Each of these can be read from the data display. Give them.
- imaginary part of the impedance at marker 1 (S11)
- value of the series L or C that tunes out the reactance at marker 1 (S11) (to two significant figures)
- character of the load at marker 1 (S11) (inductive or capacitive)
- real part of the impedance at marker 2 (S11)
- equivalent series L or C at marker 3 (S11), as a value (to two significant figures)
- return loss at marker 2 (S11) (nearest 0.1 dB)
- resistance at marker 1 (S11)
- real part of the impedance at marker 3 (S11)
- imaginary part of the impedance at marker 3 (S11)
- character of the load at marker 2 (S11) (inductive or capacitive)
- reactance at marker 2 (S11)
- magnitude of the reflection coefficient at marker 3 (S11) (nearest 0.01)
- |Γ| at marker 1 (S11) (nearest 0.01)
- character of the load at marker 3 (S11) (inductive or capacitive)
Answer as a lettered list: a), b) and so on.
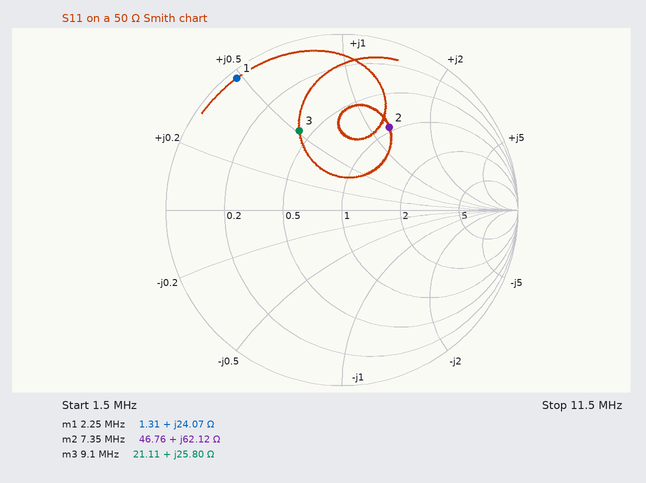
a) +24.07 Ω
b) 2.9 nF
c) inductive
d) 46.76 Ω
e) 450 nH
f) 5.3 dB
g) 1.31 Ω
h) 21.11 Ω
i) +25.80 Ω
j) inductive
k) +62.12 Ω
l) 0.51
m) 0.96
n) inductive
